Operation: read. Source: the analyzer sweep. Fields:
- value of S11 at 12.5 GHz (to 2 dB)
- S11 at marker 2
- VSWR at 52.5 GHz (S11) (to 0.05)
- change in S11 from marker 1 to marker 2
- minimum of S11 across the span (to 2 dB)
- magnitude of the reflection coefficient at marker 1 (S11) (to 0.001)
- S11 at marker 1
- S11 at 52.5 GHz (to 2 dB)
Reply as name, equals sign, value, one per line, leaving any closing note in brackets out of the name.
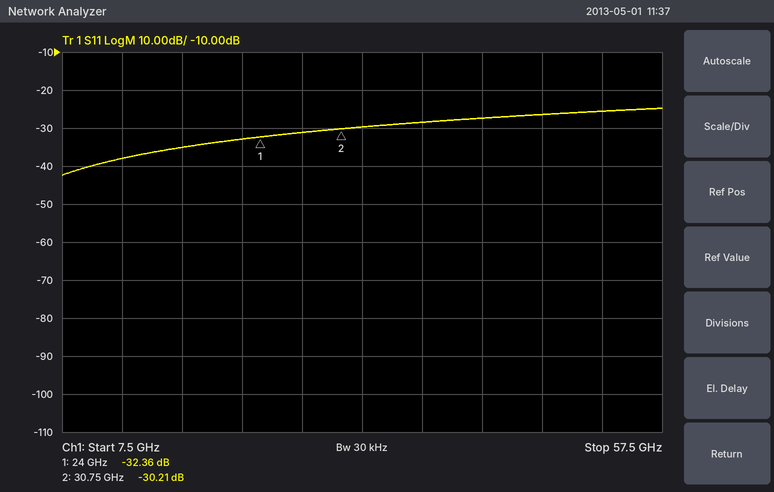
value of S11 at 12.5 GHz = -38 dB
S11 at marker 2 = -30.21 dB
VSWR at 52.5 GHz (S11) = 1.10
change in S11 from marker 1 to marker 2 = 2.15 dB
minimum of S11 across the span = -42 dB
magnitude of the reflection coefficient at marker 1 (S11) = 0.024
S11 at marker 1 = -32.36 dB
S11 at 52.5 GHz = -26 dB
